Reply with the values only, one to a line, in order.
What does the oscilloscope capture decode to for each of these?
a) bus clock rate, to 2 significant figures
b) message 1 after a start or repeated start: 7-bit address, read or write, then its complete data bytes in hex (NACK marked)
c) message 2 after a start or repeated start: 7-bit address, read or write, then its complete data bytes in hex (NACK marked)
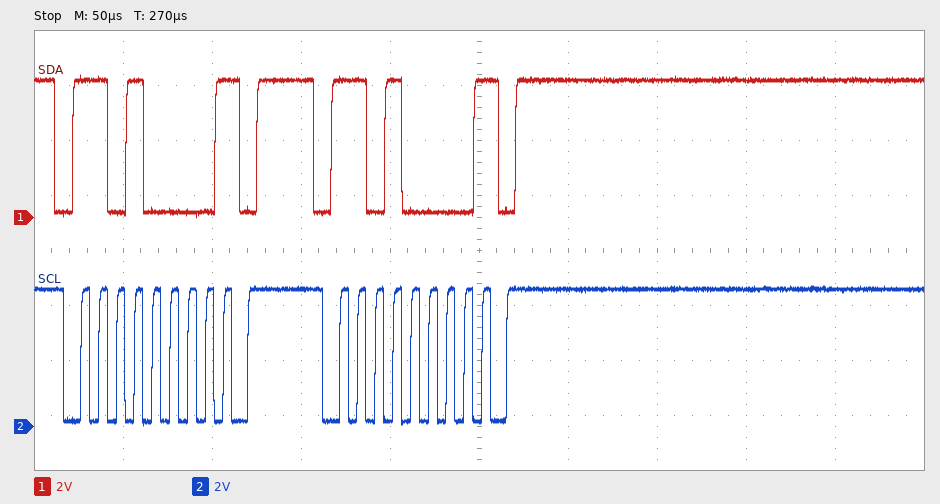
100 kHz
0x68 write NACK
0x68 write NACK
